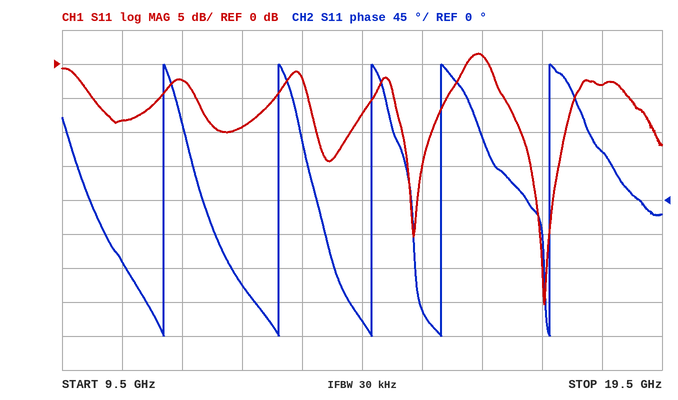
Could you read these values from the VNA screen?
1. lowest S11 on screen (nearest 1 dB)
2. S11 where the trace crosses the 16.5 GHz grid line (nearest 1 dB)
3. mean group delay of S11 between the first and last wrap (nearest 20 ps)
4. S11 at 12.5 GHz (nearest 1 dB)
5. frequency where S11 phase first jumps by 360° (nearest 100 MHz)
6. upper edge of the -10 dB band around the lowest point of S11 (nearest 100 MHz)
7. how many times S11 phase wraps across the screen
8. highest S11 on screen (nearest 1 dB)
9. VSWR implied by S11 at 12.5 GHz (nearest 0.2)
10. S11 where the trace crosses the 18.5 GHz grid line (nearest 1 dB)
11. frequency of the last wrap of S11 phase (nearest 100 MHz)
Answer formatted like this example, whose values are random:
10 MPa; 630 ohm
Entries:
-35 dB; 1 dB; 620 ps; -9 dB; 11.2 GHz; 17.9 GHz; 5; 2 dB; 2.0; -3 dB; 17.6 GHz
